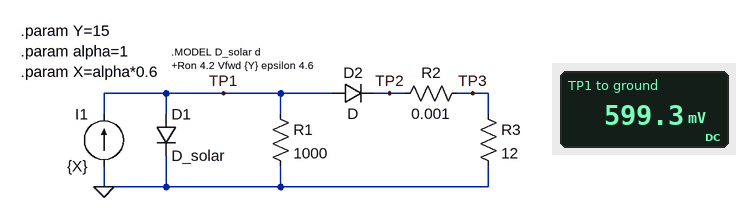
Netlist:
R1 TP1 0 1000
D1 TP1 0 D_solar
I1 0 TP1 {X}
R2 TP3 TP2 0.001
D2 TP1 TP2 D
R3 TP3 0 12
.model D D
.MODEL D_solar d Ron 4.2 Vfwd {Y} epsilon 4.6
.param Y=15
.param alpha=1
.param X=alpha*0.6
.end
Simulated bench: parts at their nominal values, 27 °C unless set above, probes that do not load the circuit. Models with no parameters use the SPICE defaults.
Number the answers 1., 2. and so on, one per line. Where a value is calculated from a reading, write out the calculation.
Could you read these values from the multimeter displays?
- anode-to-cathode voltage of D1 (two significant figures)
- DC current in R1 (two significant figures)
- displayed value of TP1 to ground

1. 599.3 mV = 600 mV
2. (599.3 mV) / 1 kΩ = 600 µA
3. 599.3 mV
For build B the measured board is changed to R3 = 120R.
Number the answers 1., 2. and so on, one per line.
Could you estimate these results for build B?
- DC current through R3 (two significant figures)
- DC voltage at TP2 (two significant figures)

1. 80 µA
2. 9.6 mV
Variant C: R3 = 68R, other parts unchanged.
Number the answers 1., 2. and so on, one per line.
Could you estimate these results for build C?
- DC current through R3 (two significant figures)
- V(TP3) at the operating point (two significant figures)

1. 91 µA
2. 6.2 mV
